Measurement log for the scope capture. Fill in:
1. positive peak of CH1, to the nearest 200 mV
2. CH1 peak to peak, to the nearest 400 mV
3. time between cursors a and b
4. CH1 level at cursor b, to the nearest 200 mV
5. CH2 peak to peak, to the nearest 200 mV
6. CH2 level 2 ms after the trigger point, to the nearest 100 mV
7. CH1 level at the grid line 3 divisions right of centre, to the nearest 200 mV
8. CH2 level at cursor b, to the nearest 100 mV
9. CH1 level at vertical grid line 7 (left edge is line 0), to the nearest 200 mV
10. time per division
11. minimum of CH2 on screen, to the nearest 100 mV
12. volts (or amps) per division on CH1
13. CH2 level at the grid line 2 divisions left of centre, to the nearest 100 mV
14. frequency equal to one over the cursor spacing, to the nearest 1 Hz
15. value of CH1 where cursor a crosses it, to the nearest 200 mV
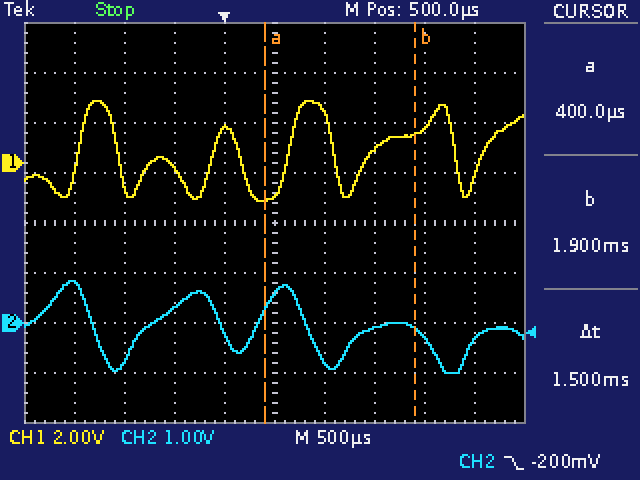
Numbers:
2.4 V
4.0 V
1.5 ms
1.2 V
1.8 V
-300 mV
1.4 V
-100 mV
600 mV
500 µs
-1.0 V
2 V
300 mV
667 Hz
-1.4 V
